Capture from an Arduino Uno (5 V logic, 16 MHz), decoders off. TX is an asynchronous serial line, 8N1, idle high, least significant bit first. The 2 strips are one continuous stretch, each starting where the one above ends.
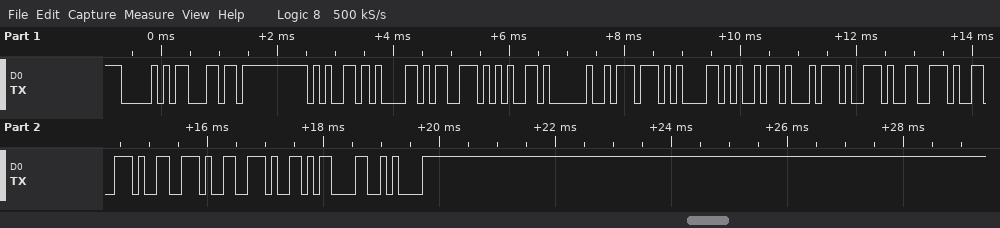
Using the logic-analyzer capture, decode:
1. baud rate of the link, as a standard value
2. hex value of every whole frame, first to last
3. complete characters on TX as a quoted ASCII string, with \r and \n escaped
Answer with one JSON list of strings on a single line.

["9600 baud", "50 6C 65 61 73 65 20 77 61 69 74 2E 2E 2E 2E 2E 0D 0A", "\"Please wait.....\\r\\n\""]
